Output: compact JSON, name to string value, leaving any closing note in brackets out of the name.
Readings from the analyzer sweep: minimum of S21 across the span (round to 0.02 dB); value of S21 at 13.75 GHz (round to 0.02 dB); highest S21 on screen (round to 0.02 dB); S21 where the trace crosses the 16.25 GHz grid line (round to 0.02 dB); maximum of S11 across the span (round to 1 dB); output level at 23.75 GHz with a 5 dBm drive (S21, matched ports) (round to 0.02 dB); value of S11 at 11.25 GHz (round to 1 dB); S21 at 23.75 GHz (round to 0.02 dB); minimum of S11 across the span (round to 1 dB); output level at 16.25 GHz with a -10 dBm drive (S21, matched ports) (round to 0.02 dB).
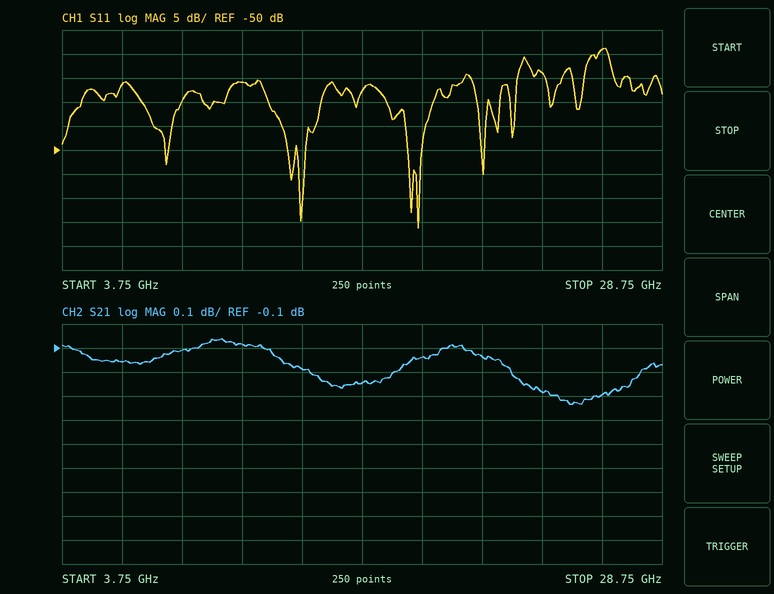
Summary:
{"minimum of S21 across the span": "-0.34 dB", "value of S21 at 13.75 GHz": "-0.18 dB", "highest S21 on screen": "-0.06 dB", "S21 where the trace crosses the 16.25 GHz grid line": "-0.24 dB", "maximum of S11 across the span": "-29 dB", "output level at 23.75 GHz with a 5 dBm drive (S21, matched ports)": "4.72 dBm", "value of S11 at 11.25 GHz": "-36 dB", "S21 at 23.75 GHz": "-0.28 dB", "minimum of S11 across the span": "-66 dB", "output level at 16.25 GHz with a -10 dBm drive (S21, matched ports)": "-10.24 dBm"}
